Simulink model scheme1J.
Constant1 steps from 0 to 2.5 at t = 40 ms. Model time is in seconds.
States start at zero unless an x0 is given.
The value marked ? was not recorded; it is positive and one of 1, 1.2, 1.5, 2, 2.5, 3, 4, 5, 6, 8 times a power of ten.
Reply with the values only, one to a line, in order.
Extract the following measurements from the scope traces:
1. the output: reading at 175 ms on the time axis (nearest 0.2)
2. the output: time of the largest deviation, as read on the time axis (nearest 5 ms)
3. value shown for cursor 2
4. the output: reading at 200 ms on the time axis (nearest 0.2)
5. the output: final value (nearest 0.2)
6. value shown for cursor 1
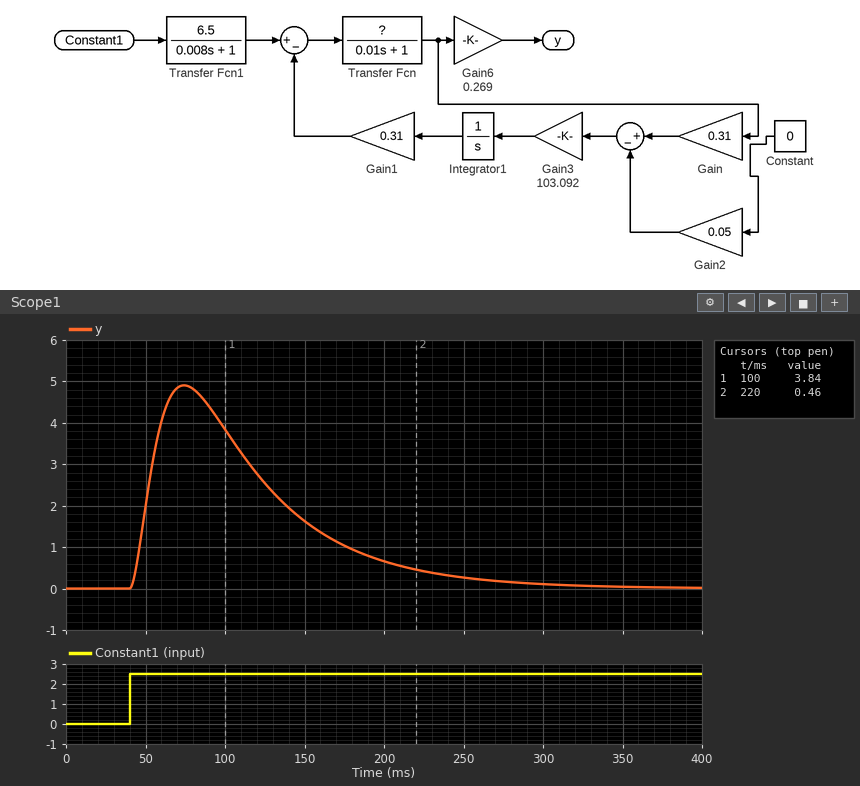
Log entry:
1.0
75 ms
0.46
0.6
0.0
3.84
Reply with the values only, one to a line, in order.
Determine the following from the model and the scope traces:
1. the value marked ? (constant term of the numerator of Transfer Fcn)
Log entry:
1.5
